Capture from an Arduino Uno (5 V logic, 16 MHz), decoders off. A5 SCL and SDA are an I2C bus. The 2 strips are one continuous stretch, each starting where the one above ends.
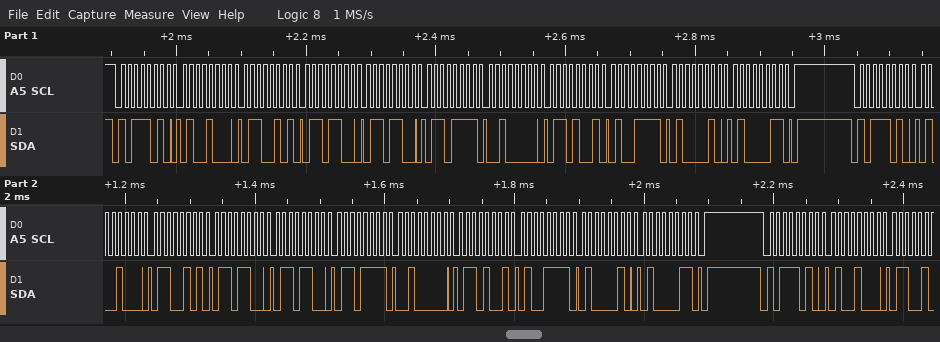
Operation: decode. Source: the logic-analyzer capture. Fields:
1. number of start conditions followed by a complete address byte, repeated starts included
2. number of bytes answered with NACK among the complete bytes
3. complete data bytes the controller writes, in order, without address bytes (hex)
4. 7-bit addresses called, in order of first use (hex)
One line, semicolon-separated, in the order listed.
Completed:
3; 0; 48 65 6C 6C 6F 20 69 4F 42 43 48 65 6C 6C 6F 20 69 4F 42 43 48; 0x5D
